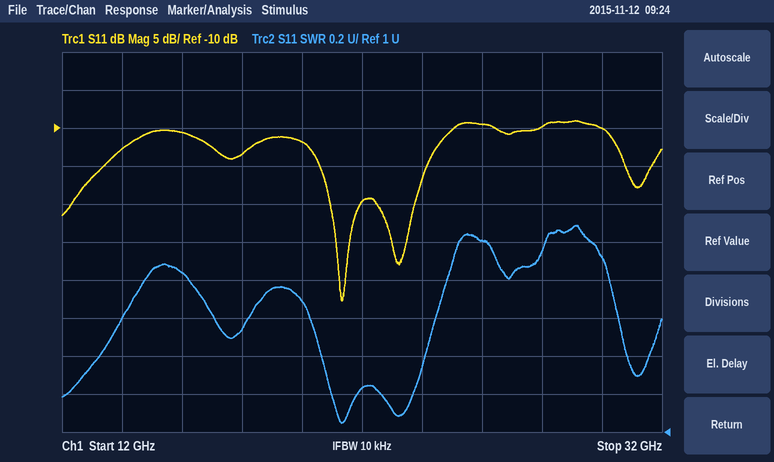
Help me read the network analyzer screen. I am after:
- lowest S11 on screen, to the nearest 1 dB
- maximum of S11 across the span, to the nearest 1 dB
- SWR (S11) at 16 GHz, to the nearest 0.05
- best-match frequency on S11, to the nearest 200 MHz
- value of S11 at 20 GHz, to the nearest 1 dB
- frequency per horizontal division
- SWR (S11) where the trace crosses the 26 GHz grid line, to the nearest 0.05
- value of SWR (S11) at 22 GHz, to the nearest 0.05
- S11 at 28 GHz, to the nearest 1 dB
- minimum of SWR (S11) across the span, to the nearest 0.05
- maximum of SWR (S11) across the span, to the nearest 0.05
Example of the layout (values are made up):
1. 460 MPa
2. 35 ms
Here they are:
1. -33 dB
2. -9 dB
3. 1.85
4. 21.4 GHz
5. -12 dB
6. 2 GHz
7. 2.00
8. 1.25
9. -10 dB
10. 1.05
11. 2.10
